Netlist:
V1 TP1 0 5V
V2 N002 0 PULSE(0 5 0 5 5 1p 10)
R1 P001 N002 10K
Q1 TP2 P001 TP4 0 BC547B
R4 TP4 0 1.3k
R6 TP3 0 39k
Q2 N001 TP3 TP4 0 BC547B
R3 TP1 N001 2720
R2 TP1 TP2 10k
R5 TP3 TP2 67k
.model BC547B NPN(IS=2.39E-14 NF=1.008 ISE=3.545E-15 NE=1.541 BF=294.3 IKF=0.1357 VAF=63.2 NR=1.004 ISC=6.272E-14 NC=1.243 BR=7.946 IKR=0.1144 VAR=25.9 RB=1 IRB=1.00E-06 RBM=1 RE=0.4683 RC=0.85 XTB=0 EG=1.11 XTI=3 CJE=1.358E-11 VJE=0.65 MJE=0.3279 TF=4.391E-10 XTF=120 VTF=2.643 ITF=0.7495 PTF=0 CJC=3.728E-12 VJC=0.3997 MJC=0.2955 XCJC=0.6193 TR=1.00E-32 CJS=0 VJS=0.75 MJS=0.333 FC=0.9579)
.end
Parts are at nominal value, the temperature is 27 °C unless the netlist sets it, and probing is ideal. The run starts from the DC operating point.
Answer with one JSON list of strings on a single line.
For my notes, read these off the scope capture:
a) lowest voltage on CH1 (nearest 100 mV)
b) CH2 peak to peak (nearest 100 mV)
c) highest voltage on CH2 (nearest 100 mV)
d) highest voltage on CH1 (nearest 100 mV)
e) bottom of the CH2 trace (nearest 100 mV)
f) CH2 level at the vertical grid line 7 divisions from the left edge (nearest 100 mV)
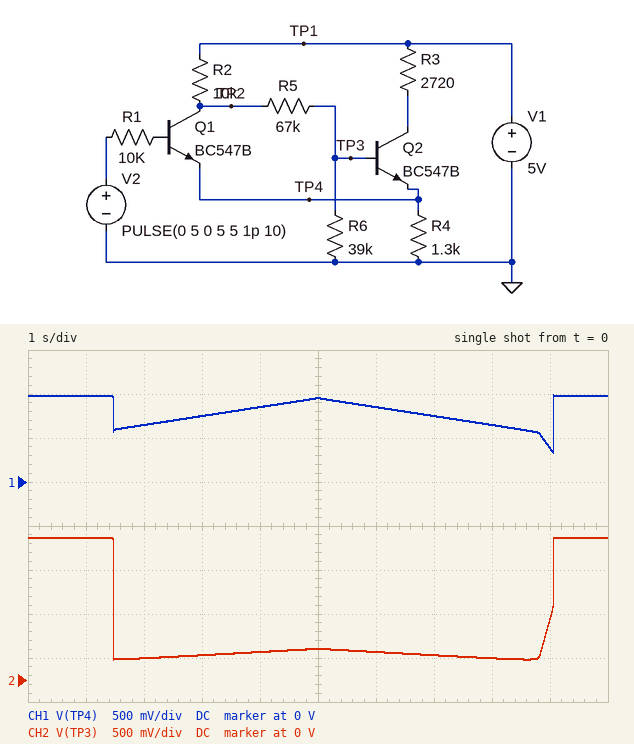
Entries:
["300 mV", "1.4 V", "1.6 V", "1.0 V", "200 mV", "300 mV"]
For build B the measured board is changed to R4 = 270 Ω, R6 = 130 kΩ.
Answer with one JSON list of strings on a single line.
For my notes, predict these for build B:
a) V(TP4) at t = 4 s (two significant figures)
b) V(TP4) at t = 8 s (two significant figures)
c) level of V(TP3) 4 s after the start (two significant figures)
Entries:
["210 mV", "160 mV", "150 mV"]
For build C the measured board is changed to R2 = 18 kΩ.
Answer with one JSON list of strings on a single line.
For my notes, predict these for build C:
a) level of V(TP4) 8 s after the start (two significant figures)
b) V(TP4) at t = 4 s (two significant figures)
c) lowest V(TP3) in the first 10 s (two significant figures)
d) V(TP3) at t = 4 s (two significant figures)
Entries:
["440 mV", "650 mV", "140 mV", "240 mV"]
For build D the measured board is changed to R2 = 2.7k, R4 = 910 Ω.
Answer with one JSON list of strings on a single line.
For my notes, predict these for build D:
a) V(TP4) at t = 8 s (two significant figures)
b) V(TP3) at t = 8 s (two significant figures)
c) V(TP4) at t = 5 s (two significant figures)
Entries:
["1.2 V", "490 mV", "1.4 V"]
